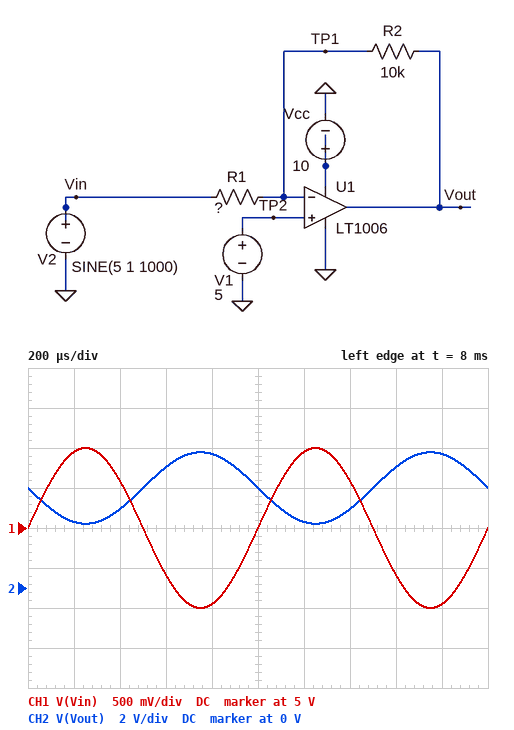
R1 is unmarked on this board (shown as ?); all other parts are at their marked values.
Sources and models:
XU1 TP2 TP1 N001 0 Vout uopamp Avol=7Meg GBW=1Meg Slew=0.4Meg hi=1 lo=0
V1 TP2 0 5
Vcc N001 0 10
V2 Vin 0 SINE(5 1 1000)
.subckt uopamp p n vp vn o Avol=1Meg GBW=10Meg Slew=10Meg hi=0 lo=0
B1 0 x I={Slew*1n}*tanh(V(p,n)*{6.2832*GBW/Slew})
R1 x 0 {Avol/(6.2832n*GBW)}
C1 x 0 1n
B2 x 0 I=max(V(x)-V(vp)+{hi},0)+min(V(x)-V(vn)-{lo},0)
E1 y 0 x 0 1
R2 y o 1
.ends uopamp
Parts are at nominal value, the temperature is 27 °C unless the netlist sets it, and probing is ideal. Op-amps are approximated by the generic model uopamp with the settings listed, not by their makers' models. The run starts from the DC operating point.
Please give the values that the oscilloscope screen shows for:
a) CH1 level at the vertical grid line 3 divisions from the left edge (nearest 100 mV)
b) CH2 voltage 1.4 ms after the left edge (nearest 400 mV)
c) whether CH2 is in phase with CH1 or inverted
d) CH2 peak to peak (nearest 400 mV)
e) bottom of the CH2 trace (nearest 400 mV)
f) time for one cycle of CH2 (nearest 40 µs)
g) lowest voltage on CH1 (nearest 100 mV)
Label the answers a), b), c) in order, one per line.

a) 4.4 V
b) 4.0 V
c) inverted
d) 3.6 V
e) 3.2 V
f) 1.00 ms
g) 4.0 V
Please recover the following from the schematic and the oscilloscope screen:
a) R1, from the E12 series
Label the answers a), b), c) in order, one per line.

a) 5.6 kΩ
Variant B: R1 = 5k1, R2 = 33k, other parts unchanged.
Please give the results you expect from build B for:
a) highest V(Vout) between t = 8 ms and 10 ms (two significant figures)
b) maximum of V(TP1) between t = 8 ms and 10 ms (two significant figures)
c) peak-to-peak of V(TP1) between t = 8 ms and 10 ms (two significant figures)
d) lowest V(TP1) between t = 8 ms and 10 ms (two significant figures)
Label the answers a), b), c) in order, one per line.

a) 9.0 V
b) 5.2 V
c) 530 mV
d) 4.7 V
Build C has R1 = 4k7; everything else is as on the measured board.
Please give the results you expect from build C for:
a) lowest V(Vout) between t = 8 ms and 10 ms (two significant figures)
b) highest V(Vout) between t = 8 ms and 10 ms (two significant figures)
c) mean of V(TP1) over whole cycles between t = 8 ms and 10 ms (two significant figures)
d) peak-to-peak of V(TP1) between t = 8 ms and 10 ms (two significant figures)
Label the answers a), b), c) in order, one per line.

a) 2.9 V
b) 7.1 V
c) 5.0 V
d) 4.3 mV
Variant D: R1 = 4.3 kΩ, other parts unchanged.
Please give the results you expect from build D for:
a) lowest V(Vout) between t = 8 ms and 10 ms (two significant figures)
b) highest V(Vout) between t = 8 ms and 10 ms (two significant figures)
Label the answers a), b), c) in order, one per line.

a) 2.7 V
b) 7.3 V
